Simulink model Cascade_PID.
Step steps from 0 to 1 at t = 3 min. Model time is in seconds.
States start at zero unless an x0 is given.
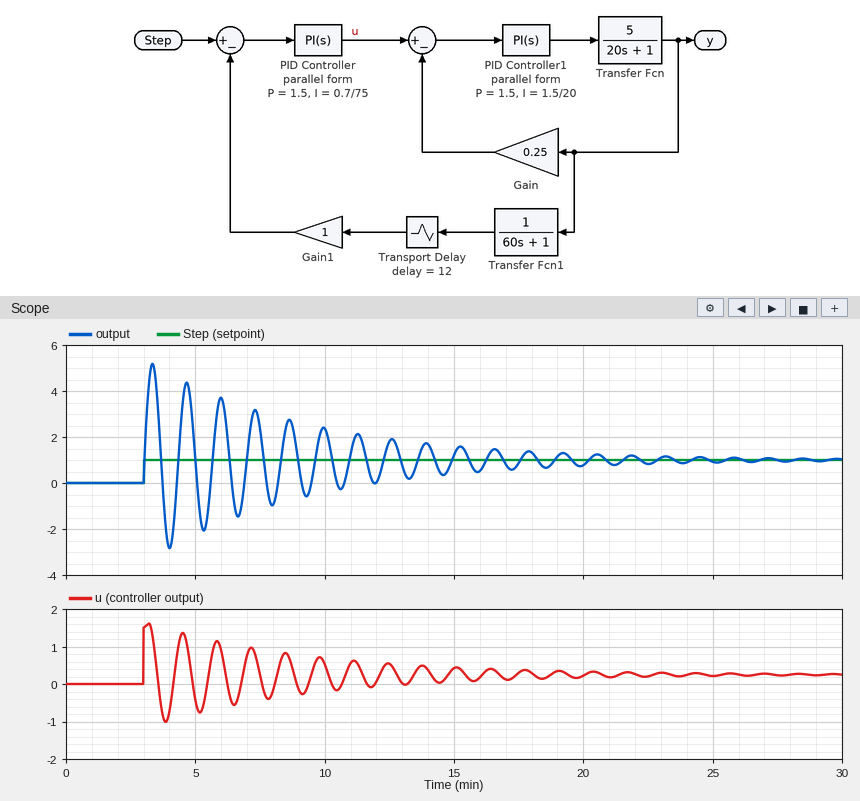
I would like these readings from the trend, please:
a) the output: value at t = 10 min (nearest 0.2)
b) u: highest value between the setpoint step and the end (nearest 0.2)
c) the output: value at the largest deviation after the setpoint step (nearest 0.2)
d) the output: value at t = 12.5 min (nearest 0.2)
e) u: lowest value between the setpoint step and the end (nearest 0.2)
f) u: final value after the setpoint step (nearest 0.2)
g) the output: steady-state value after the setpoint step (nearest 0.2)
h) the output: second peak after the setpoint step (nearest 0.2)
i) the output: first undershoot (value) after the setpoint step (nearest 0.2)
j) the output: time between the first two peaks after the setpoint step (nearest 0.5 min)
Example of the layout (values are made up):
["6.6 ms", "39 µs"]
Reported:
["2.4", "1.6", "5.2", "1.8", "-1.0", "0.2", "1.0", "4.4", "-2.8", "1.5 min"]
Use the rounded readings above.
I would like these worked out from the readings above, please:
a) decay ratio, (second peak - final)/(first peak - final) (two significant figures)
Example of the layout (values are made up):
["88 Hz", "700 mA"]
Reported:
["0.81"]
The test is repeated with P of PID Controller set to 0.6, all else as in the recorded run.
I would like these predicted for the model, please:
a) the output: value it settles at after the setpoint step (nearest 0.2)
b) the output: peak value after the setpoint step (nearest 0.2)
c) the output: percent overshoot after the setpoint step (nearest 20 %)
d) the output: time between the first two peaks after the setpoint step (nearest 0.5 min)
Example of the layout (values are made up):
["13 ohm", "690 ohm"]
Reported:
["1.0", "2.6", "160 %", "2.0 min"]
